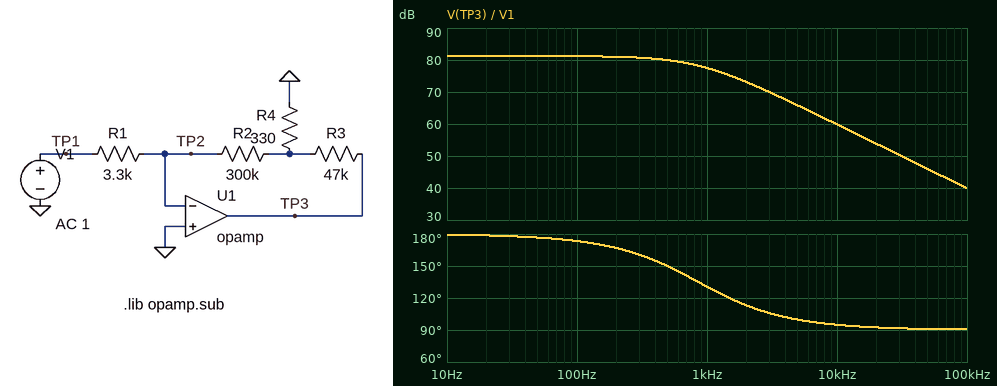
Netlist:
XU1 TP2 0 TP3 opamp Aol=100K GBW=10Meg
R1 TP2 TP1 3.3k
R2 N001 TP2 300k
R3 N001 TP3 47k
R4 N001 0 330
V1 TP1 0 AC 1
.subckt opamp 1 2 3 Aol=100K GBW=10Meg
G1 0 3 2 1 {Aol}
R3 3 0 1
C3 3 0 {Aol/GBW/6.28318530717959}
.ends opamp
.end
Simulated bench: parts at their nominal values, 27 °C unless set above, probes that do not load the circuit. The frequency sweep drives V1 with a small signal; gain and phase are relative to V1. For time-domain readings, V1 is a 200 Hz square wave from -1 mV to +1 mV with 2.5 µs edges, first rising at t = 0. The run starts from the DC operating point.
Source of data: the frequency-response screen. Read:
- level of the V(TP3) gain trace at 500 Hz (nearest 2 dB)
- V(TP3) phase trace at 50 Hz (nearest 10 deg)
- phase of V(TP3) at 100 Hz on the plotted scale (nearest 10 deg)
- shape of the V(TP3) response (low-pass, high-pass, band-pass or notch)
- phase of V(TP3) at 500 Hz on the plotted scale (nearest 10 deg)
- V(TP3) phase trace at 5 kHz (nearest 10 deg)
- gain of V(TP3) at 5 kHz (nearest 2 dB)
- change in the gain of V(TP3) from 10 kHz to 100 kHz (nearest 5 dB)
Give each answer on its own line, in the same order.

80 dB
180 deg
170 deg
low-pass
150 deg
100 deg
66 dB
-20 dB
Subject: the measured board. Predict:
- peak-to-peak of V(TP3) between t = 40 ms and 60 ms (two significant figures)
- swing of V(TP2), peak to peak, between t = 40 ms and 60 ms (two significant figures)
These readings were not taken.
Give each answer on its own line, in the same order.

23 V
3.7 mV
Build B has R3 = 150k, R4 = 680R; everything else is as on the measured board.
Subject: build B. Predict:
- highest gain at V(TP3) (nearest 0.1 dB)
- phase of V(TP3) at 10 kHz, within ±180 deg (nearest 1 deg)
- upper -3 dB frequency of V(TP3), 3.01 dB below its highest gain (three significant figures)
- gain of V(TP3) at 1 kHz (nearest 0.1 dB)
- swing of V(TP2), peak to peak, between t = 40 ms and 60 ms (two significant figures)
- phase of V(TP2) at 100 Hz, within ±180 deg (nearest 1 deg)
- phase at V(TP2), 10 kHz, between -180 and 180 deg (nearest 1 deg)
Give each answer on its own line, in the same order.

84.5 dB
93 deg
590 Hz
78.6 dB
3.6 mV
35 deg
3 deg
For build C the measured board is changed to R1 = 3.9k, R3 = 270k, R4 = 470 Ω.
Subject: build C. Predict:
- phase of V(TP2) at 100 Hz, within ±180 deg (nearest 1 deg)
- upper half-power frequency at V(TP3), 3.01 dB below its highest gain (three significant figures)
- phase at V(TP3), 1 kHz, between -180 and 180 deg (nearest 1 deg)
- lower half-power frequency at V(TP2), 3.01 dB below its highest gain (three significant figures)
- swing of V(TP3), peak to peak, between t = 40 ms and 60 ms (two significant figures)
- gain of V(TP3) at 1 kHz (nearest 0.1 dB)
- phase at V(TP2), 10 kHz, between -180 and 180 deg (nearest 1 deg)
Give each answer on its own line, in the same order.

28 deg
323 Hz
108 deg
290 Hz
60 V
79.5 dB
1 deg
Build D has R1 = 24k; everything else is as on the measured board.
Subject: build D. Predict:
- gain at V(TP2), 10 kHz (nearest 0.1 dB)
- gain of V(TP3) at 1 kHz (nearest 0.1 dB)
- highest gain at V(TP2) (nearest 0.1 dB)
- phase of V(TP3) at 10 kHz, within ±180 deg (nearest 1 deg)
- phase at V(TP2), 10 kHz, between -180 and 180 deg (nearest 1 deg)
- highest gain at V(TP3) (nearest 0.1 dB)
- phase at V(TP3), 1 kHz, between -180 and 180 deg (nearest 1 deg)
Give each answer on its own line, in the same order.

-1.7 dB
64.8 dB
-0.7 dB
118 deg
27 deg
64.9 dB
169 deg
